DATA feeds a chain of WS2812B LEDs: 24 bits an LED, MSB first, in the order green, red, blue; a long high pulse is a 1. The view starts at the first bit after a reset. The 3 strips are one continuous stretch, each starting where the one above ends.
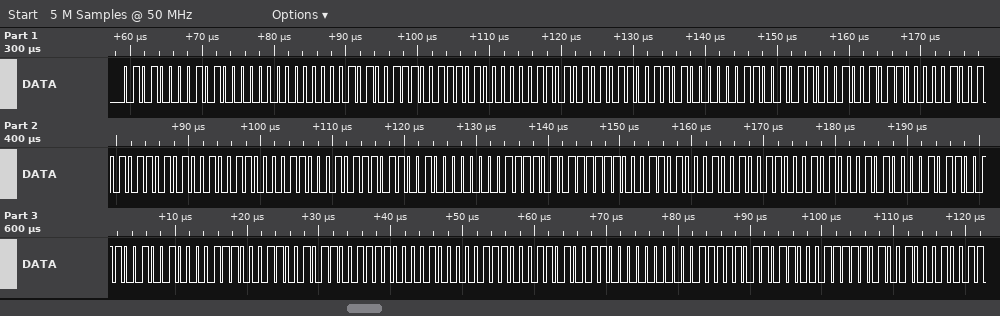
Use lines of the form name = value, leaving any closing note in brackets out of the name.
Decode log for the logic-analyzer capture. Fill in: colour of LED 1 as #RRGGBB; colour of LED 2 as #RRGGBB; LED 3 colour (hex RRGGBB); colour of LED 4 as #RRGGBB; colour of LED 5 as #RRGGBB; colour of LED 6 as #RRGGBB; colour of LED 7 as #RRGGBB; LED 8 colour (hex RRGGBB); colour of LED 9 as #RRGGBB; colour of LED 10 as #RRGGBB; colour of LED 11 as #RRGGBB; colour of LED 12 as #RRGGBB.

colour of LED 1 as #RRGGBB = #A05000
colour of LED 2 as #RRGGBB = #9D5303
LED 3 colour = #9A5506
colour of LED 4 as #RRGGBB = #965809
colour of LED 5 as #RRGGBB = #935A0C
colour of LED 6 as #RRGGBB = #905D0F
colour of LED 7 as #RRGGBB = #8D5F12
LED 8 colour = #8A6216
colour of LED 9 as #RRGGBB = #876419
colour of LED 10 as #RRGGBB = #84671C
colour of LED 11 as #RRGGBB = #80691F
colour of LED 12 as #RRGGBB = #7D6C22
